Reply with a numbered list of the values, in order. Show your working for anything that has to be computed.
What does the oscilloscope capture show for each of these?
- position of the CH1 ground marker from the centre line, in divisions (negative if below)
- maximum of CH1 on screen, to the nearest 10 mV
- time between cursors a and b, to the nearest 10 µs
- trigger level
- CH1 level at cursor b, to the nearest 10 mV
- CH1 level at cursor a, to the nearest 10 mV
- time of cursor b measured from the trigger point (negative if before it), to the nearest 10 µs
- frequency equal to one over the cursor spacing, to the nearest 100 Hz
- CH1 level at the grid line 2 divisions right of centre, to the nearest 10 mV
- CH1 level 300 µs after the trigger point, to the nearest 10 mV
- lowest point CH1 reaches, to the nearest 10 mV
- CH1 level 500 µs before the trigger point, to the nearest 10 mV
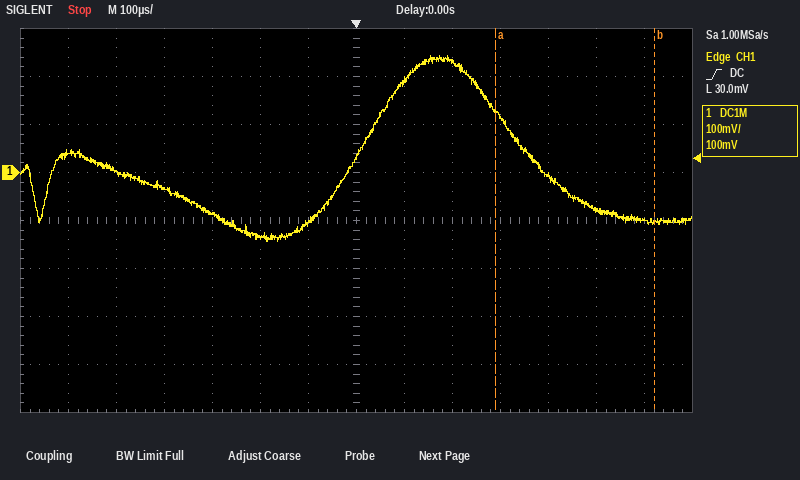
1. +1.0 div
2. 240 mV
3. 330 µs
4. 30.0 mV
5. -100 mV
6. 130 mV
7. +620 µs
8. 1 / 330 µs ≈ 3.0 kHz
9. 230 mV
10. 120 mV
11. -140 mV
12. 0 mV
